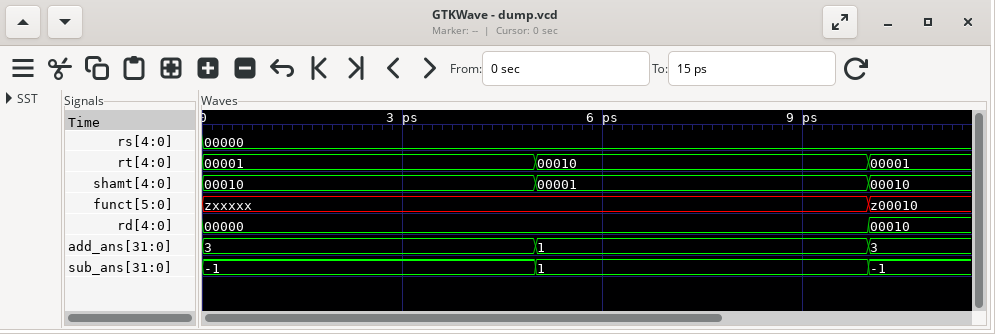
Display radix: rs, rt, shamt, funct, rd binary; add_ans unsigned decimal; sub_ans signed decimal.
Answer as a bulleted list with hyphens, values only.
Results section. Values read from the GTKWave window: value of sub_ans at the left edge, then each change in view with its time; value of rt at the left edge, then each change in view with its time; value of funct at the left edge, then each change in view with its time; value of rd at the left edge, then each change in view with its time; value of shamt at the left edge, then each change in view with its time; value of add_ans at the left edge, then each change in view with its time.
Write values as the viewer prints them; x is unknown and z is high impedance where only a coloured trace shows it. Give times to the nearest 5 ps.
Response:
- -1, 1 at 5 ps, -1 at 10 ps
- 00001, 00010 at 5 ps, 00001 at 10 ps
- zxxxxx, z00010 at 10 ps
- 00000, 00010 at 10 ps
- 00010, 00001 at 5 ps, 00010 at 10 ps
- 3, 1 at 5 ps, 3 at 10 ps
